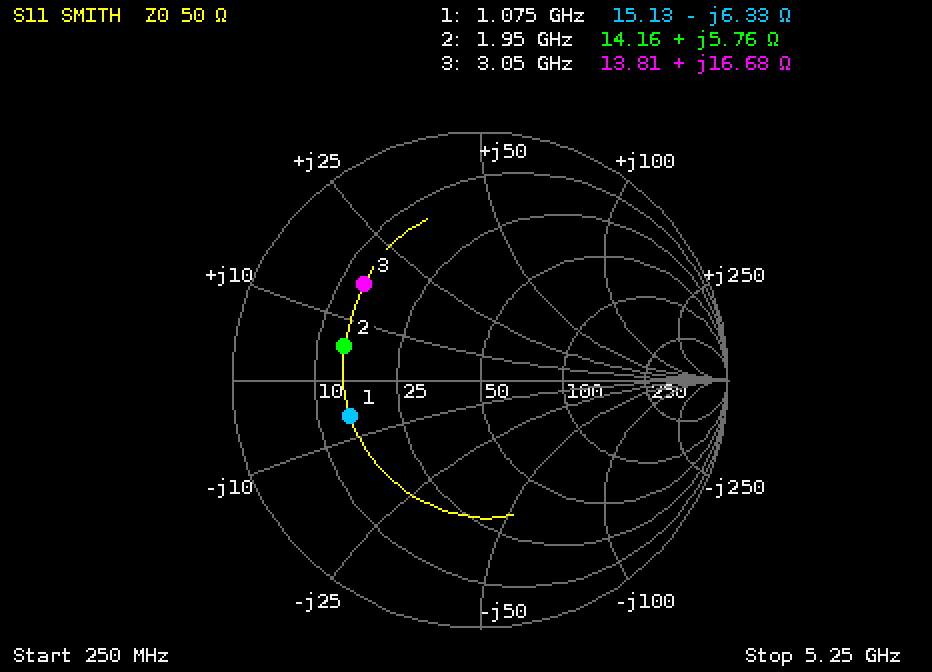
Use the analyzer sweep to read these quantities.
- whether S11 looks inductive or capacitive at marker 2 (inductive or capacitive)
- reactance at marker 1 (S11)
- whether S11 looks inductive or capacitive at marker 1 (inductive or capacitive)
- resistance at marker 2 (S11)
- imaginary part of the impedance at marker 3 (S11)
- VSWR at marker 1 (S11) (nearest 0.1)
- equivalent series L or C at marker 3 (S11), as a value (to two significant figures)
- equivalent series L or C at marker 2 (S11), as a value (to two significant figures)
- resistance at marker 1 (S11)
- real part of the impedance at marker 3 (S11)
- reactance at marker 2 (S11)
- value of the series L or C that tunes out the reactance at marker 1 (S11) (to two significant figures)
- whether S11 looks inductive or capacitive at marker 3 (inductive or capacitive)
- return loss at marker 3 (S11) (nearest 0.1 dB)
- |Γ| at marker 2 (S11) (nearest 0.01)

inductive
-6.33 Ω
capacitive
14.16 Ω
+16.68 Ω
3.4
870 pH
470 pH
15.13 Ω
13.81 Ω
+5.76 Ω
940 pH
inductive
4.4 dB
0.56
